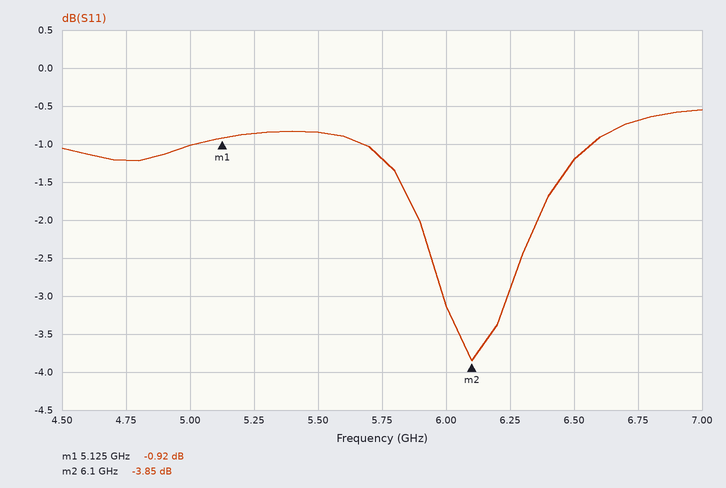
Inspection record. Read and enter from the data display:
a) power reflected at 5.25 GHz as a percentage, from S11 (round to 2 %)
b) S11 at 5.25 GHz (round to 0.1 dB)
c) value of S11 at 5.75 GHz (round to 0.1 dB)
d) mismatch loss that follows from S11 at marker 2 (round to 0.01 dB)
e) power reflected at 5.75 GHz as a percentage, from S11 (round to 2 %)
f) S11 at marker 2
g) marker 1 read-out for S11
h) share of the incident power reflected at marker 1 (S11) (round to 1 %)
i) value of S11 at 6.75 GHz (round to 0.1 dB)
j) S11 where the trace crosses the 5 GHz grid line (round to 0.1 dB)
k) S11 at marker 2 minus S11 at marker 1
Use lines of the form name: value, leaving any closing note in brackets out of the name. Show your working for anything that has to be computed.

power reflected at 5.25 GHz as a percentage, from S11: 10^(-0.9/10) ≈ 81.3 %, so 82 % to the nearest 2 %
S11 at 5.25 GHz: -0.9 dB
value of S11 at 5.75 GHz: -1.2 dB
mismatch loss that follows from S11 at marker 2: −10 log10(1 − 10^(-3.85/10)) ≈ 2.31 dB
power reflected at 5.75 GHz as a percentage, from S11: 10^(-1.2/10) ≈ 76 %
S11 at marker 2: -3.85 dB
marker 1 read-out for S11: -0.92 dB
share of the incident power reflected at marker 1 (S11): 10^(-0.92/10) ≈ 81 %
value of S11 at 6.75 GHz: -0.7 dB
S11 where the trace crosses the 5 GHz grid line: -1.0 dB
S11 at marker 2 minus S11 at marker 1: -3.85 − (-0.92) = -2.93 dB
